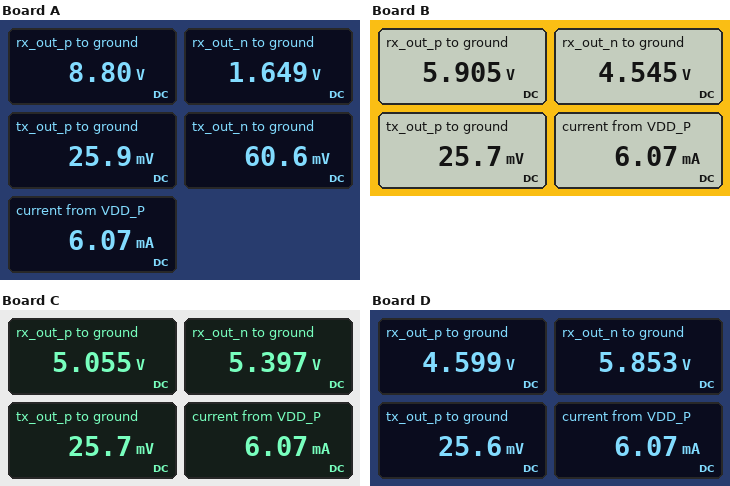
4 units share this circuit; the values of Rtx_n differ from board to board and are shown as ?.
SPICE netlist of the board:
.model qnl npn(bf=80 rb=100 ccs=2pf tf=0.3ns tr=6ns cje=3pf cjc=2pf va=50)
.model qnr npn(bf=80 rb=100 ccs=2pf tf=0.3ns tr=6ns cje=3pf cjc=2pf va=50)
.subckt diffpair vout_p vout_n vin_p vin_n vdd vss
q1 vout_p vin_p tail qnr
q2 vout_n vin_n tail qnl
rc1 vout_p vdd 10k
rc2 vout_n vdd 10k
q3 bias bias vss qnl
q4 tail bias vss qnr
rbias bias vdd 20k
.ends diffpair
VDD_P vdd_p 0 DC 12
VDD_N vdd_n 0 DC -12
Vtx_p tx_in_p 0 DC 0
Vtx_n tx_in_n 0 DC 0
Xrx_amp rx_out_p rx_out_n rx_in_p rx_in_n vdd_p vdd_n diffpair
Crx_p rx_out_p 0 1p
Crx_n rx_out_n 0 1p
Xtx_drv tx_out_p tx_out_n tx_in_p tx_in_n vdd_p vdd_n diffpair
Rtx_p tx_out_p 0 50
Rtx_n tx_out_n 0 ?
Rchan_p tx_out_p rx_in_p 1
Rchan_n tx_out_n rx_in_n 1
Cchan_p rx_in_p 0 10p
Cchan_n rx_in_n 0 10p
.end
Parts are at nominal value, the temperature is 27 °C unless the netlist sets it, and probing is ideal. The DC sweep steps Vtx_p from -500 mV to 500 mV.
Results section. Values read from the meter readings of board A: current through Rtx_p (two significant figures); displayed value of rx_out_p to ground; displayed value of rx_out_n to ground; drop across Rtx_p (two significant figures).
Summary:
520 µA
8.80 V
1.649 V
26 mV
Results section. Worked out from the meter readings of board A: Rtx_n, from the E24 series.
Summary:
120 Ω
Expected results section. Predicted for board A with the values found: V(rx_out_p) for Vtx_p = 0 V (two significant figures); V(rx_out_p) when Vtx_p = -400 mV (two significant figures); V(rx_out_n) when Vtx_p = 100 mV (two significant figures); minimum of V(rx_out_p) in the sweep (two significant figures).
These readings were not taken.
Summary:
8.8 V
-590 mV
-590 mV
-590 mV
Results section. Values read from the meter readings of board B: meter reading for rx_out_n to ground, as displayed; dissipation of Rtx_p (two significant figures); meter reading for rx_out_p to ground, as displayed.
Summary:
4.545 V
13 µW
5.905 V
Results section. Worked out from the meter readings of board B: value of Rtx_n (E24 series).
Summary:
62 Ω
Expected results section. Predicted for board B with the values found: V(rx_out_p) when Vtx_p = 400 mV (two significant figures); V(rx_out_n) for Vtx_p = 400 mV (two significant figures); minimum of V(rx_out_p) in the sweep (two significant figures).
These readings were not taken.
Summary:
11 V
-590 mV
-390 mV
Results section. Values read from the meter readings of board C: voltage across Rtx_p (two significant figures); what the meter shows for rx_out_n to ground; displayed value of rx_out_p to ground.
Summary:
26 mV
5.397 V
5.055 V
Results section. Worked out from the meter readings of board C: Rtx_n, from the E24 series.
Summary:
47 Ω
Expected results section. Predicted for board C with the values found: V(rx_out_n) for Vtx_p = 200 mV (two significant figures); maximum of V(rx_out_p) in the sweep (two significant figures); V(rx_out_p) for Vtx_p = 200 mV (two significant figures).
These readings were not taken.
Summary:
-180 mV
11 V
11 V
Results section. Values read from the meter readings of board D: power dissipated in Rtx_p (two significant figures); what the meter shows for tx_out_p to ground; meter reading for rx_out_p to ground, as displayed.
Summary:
13 µW
25.6 mV
4.599 V
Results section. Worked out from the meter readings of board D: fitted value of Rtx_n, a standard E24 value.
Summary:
39 Ω
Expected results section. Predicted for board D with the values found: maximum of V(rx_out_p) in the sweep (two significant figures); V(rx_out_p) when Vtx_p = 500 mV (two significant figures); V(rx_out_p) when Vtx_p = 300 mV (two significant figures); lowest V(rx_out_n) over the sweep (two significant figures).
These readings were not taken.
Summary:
10 V
10 V
10 V
270 mV
